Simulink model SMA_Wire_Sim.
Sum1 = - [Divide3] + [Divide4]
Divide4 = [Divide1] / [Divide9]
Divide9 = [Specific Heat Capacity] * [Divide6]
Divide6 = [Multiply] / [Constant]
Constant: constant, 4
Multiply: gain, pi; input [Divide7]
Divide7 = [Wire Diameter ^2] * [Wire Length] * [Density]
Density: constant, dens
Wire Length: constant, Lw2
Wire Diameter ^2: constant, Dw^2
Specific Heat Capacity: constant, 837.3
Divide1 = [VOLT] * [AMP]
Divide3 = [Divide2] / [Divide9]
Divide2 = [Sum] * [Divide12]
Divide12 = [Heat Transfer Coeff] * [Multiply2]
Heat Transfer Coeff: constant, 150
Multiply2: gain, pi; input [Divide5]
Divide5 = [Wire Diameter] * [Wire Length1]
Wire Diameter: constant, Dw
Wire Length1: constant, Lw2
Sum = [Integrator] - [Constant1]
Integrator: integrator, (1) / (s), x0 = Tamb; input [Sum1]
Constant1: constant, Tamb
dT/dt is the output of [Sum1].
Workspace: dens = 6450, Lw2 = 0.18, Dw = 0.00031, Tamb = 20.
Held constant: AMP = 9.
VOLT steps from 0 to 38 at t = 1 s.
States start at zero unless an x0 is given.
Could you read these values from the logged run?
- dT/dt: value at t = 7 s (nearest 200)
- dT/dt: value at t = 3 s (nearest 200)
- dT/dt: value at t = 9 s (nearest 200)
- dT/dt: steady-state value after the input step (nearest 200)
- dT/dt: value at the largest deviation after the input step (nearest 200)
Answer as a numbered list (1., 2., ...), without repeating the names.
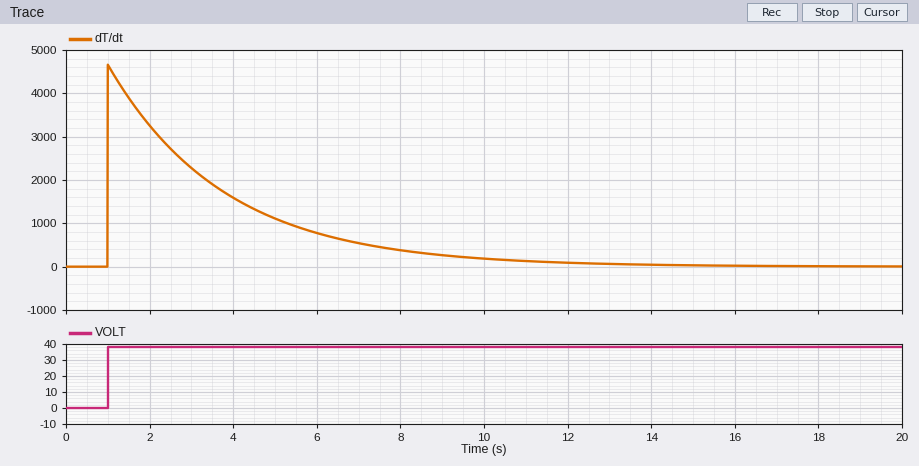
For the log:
1. 600
2. 2200
3. 200
4. 0
5. 4600
